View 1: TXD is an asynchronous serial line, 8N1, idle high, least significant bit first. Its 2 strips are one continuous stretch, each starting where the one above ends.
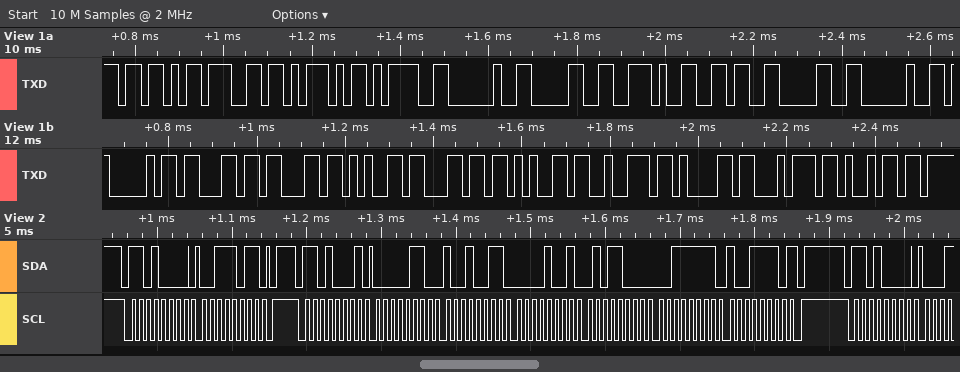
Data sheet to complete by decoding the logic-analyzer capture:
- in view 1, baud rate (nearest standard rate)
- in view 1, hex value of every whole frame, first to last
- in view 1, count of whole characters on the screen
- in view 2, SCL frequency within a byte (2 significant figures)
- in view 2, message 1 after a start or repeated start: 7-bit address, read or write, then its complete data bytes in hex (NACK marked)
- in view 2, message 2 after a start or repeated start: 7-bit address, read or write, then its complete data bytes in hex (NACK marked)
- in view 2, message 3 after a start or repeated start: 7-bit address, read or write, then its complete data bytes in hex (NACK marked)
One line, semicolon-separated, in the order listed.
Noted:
57600 baud; 5B 67 5D 3D 20 30 2E 36 30 20 41 63 63 65 6C 65 72 61 74 69; 20; 100 kHz; 0x68 write: 3B; 0x68 read: 06 93 09 58 3F 9E NACK; 0x68 write
